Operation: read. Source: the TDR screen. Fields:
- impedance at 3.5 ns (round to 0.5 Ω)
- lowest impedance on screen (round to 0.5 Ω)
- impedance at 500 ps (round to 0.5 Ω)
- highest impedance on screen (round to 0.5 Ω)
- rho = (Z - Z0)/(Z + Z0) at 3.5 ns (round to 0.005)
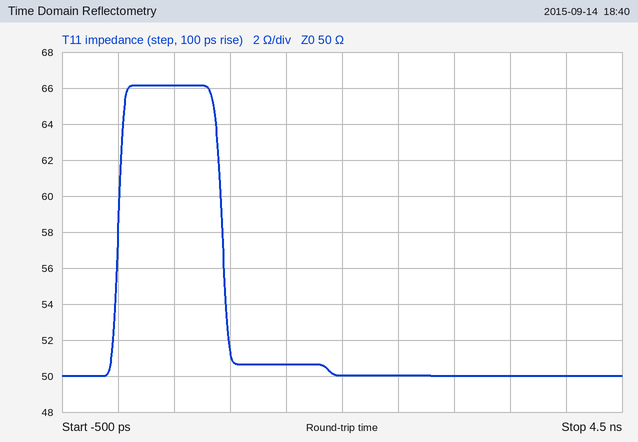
50.0 Ω
50.0 Ω
66.0 Ω
66.0 Ω
0.000
